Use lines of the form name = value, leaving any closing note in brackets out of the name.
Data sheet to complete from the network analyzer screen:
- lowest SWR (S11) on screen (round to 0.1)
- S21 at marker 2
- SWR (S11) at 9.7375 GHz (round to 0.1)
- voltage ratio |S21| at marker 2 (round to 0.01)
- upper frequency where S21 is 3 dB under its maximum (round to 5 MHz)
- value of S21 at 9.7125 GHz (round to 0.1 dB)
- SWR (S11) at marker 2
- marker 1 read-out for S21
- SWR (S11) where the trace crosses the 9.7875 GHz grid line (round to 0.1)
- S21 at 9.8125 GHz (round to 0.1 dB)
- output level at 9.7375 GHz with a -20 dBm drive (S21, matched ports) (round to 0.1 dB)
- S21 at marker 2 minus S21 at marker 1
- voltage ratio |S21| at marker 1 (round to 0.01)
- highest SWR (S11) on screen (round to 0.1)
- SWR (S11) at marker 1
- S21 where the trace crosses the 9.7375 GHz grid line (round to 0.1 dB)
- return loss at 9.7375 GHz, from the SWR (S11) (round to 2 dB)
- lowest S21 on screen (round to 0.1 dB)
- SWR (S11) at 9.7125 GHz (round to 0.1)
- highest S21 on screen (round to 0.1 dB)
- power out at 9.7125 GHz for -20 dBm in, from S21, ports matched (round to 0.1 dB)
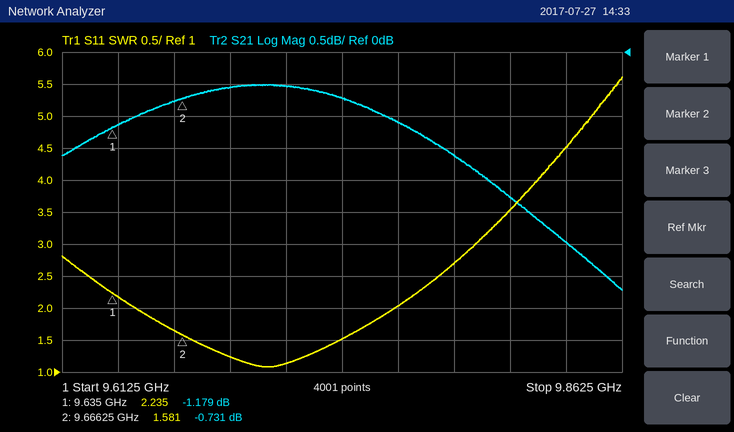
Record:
lowest SWR (S11) on screen = 1.1
S21 at marker 2 = -0.731 dB
SWR (S11) at 9.7375 GHz = 1.5
voltage ratio |S21| at marker 2 = 0.92
upper frequency where S21 is 3 dB under its maximum = 9.855 GHz
value of S21 at 9.7125 GHz = -0.5 dB
SWR (S11) at marker 2 = 1.581
marker 1 read-out for S21 = -1.179 dB
SWR (S11) where the trace crosses the 9.7875 GHz grid line = 2.7
S21 at 9.8125 GHz = -2.3 dB
output level at 9.7375 GHz with a -20 dBm drive (S21, matched ports) = -20.7 dBm
S21 at marker 2 minus S21 at marker 1 = 0.448 dB
voltage ratio |S21| at marker 1 = 0.87
highest SWR (S11) on screen = 5.6
SWR (S11) at marker 1 = 2.235
S21 where the trace crosses the 9.7375 GHz grid line = -0.7 dB
return loss at 9.7375 GHz, from the SWR (S11) = 14 dB
lowest S21 on screen = -3.7 dB
SWR (S11) at 9.7125 GHz = 1.1
highest S21 on screen = -0.5 dB
power out at 9.7125 GHz for -20 dBm in, from S21, ports matched = -20.5 dBm
